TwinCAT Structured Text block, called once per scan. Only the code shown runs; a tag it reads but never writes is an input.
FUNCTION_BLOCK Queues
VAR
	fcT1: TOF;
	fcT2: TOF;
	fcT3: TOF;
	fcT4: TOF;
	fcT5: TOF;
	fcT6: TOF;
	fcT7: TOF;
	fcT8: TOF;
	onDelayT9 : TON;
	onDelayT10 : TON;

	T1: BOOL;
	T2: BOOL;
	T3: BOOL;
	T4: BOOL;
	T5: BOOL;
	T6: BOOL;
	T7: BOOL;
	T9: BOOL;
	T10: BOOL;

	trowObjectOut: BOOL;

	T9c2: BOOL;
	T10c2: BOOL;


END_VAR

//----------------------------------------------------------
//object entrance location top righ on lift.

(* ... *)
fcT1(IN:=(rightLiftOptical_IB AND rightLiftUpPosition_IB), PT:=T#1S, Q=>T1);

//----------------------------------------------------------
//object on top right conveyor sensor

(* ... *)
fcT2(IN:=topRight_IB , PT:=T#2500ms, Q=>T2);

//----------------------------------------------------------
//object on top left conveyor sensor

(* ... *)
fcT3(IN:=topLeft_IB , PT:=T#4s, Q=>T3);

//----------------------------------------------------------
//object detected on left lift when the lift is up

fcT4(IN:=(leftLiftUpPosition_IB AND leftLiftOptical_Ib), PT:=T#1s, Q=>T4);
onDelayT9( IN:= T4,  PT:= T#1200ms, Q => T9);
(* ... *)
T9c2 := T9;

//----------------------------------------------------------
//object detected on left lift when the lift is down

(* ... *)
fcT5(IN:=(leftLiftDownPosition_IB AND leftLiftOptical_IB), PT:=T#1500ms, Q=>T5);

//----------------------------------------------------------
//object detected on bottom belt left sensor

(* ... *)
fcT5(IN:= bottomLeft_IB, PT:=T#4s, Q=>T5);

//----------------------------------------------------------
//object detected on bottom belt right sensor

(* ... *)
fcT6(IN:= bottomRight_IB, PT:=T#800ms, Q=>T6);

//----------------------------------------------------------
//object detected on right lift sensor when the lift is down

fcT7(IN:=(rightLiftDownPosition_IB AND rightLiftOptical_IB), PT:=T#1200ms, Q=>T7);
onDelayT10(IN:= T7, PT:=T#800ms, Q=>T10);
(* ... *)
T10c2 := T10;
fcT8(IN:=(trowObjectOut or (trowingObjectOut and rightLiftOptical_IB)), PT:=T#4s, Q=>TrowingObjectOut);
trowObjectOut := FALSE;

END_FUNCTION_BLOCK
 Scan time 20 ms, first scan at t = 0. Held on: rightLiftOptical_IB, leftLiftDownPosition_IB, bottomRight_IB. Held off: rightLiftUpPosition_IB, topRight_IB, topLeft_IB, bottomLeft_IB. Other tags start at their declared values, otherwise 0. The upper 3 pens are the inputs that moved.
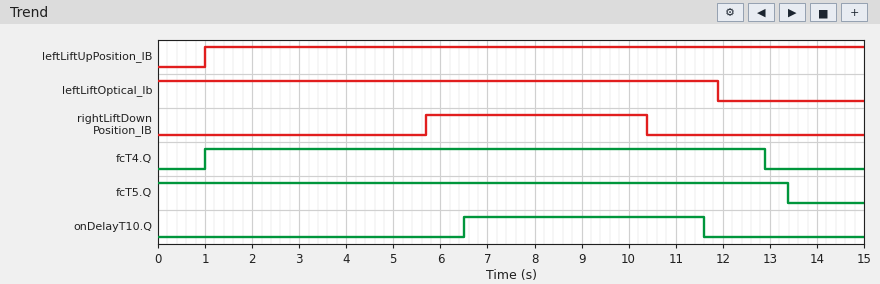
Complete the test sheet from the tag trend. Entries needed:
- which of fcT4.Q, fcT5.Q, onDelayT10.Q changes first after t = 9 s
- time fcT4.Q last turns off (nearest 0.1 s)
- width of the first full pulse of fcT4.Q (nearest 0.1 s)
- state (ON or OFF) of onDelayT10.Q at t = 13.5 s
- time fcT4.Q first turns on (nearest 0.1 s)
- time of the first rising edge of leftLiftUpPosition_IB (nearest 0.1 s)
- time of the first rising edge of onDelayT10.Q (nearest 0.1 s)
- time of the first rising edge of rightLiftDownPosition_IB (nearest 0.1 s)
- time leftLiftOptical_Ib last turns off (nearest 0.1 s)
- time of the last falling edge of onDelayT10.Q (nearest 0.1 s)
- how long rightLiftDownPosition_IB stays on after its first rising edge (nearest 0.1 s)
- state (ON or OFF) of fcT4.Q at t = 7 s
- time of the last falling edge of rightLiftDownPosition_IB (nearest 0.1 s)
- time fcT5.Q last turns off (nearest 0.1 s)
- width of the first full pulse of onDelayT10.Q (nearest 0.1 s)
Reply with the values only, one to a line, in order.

onDelayT10.Q
12.9 s
11.9 s
OFF
1.0 s
1.0 s
6.5 s
5.7 s
11.9 s
11.6 s
4.7 s
ON
10.4 s
13.4 s
5.1 s
